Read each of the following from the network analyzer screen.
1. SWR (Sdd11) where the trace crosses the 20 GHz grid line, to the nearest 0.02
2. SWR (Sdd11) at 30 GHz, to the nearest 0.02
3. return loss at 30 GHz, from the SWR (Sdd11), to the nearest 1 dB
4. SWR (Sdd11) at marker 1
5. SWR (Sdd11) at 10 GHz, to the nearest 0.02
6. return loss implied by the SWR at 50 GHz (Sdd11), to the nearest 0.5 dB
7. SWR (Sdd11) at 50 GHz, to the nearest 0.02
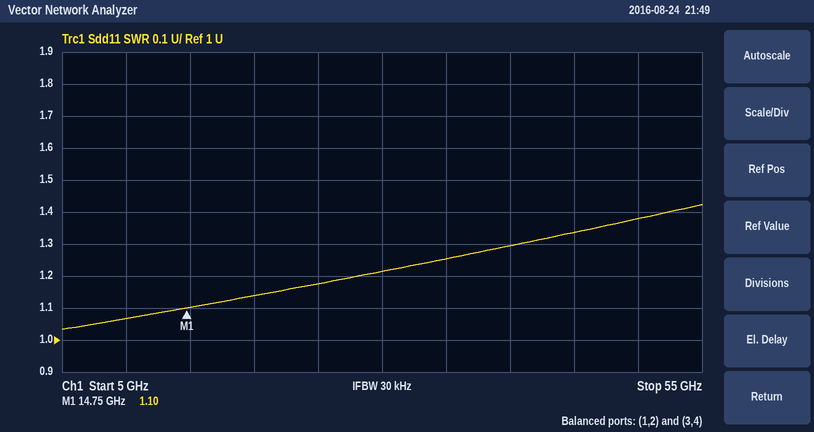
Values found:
1.14
1.22
20 dB
1.10
1.06
16.0 dB
1.38
